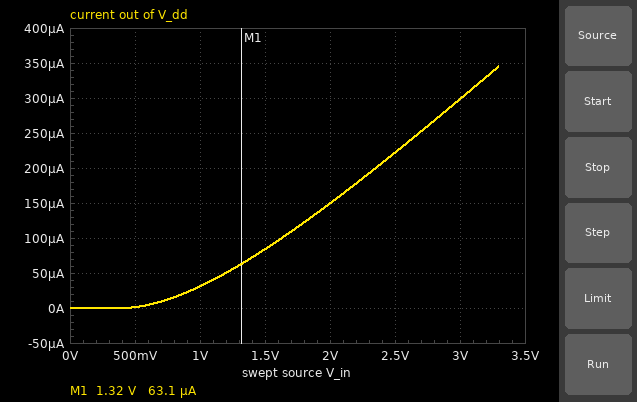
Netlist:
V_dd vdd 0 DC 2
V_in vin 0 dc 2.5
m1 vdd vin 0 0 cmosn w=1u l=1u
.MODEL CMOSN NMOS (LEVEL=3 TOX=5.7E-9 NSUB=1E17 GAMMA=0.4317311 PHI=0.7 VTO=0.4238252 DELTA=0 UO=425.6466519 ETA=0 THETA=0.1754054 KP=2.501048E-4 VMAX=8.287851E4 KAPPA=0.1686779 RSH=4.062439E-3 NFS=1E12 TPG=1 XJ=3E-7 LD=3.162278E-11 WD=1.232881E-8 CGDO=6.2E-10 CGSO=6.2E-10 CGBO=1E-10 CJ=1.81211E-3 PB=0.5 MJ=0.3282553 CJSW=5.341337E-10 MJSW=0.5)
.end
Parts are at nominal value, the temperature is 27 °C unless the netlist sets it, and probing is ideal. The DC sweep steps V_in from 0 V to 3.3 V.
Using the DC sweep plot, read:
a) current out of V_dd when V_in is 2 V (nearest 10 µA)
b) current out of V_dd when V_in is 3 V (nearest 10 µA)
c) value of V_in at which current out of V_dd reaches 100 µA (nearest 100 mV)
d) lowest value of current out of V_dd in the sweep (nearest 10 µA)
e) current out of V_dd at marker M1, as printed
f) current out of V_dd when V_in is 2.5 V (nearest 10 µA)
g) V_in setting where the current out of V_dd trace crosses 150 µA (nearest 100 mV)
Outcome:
150 µA
300 µA
1.6 V
0 A
63.1 µA
220 µA
2.0 V
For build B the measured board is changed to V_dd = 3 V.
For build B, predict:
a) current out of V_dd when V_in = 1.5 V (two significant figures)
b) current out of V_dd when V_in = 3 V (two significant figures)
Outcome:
86 µA
310 µA
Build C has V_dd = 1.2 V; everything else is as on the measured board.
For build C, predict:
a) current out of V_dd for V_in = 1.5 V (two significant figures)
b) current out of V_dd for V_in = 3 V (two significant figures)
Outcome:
82 µA
270 µA
